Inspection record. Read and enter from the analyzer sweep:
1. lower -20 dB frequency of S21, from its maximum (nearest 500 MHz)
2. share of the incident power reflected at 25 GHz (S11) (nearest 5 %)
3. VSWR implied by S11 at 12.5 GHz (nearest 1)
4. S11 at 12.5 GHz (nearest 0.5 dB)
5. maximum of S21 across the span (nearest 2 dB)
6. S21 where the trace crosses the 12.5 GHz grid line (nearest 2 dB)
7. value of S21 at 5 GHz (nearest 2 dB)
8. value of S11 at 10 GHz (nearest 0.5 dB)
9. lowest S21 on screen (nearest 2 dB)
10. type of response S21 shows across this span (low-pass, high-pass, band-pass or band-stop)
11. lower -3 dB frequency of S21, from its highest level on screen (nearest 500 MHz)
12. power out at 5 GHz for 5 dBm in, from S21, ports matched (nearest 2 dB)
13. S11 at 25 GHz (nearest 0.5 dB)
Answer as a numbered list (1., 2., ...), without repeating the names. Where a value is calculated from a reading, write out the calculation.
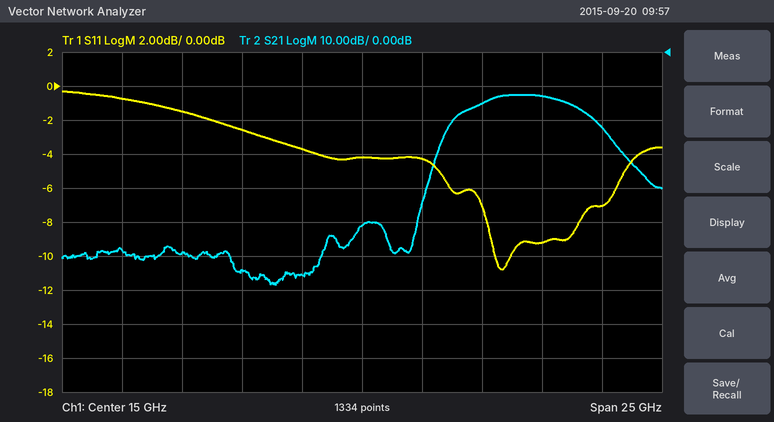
1. 18.0 GHz
2. 10^(-7/10) ≈ 20 %
3. |Γ| = 10^(-3.5/20) = 0.6683; VSWR = (1 + 0.6683)/(1 − 0.6683) ≈ 5
4. -3.5 dB
5. -12 dB
6. -66 dB
7. -58 dB
8. -2.5 dB
9. -68 dB
10. band-pass
11. 20.0 GHz
12. 5 dBm + (-58 dB) = -54 dBm
13. -7.0 dB
